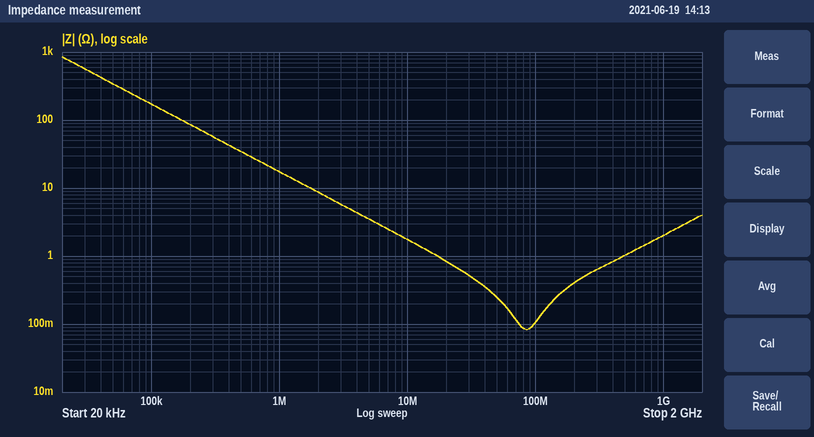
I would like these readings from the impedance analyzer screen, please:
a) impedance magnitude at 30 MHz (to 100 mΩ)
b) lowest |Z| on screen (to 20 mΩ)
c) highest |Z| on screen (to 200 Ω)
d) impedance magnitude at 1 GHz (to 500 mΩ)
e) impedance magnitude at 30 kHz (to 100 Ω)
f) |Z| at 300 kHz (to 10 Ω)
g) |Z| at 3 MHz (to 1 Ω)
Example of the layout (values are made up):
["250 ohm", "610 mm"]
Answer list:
["500 mΩ", "80 mΩ", "800 Ω", "2.0 Ω", "600 Ω", "60 Ω", "6 Ω"]
